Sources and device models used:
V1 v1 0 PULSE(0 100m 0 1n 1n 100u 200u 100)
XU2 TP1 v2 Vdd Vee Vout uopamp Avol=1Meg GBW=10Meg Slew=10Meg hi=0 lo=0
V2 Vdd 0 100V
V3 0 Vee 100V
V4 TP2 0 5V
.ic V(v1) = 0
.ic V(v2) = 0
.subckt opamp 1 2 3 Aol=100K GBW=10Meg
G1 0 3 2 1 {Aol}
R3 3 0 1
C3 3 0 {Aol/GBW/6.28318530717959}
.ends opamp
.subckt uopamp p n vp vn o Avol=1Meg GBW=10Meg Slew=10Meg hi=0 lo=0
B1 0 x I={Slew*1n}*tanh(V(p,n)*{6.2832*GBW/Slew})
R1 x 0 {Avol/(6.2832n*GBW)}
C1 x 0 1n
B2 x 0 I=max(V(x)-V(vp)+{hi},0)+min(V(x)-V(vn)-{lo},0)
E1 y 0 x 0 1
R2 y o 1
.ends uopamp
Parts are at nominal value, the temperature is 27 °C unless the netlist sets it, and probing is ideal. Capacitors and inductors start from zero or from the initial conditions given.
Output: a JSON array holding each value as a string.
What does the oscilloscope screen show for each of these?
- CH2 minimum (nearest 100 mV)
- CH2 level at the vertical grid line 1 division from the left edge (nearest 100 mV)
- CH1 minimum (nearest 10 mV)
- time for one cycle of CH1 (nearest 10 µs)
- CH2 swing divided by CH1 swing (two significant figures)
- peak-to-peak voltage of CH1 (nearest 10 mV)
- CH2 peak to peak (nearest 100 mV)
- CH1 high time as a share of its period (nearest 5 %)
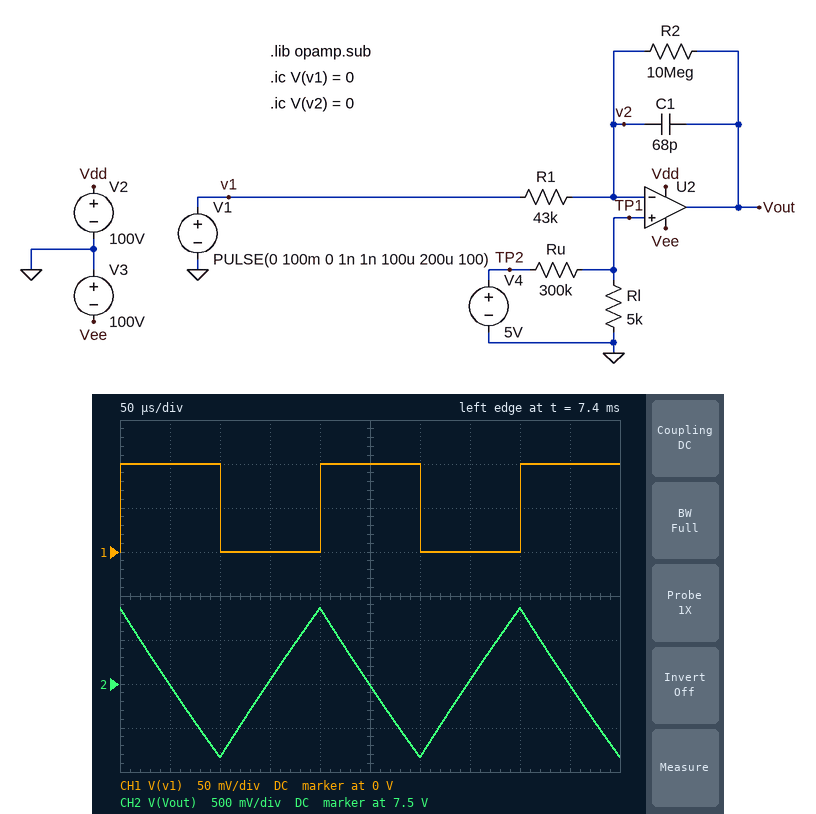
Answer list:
["6.7 V", "7.5 V", "0 V", "200 µs", "17", "100 mV", "1.7 V", "50 %"]
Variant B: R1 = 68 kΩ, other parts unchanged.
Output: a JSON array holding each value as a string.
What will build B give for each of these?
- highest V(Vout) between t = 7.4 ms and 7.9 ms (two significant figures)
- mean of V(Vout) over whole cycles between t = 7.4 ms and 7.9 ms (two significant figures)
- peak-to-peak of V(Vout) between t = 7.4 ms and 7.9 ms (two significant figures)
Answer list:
["5.3 V", "4.8 V", "1.1 V"]
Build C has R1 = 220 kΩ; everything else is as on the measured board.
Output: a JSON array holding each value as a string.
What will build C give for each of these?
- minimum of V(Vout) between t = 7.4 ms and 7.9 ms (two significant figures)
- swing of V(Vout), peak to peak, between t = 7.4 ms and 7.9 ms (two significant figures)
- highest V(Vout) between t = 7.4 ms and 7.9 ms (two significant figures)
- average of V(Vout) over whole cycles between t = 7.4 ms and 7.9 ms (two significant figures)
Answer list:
["1.4 V", "330 mV", "1.7 V", "1.5 V"]
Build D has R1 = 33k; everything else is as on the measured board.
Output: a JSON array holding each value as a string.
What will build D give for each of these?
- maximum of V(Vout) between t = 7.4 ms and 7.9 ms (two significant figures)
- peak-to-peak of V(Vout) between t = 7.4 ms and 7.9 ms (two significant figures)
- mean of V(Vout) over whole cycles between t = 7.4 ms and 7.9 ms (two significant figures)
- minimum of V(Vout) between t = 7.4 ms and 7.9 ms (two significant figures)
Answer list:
["11 V", "2.2 V", "9.8 V", "8.7 V"]
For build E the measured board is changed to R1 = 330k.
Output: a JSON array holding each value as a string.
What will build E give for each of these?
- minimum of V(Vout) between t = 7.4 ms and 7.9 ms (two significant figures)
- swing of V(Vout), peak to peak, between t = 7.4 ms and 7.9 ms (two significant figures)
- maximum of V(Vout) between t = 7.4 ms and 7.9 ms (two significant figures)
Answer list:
["940 mV", "220 mV", "1.2 V"]
